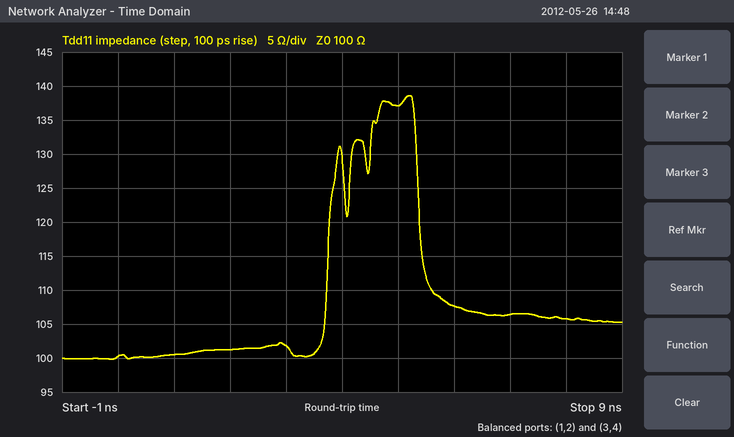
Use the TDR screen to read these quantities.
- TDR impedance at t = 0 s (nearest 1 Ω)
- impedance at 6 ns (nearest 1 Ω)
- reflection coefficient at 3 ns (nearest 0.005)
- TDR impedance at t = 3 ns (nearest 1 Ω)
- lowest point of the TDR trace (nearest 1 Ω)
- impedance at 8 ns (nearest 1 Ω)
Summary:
100 Ω
108 Ω
+0.010
102 Ω
100 Ω
106 Ω
